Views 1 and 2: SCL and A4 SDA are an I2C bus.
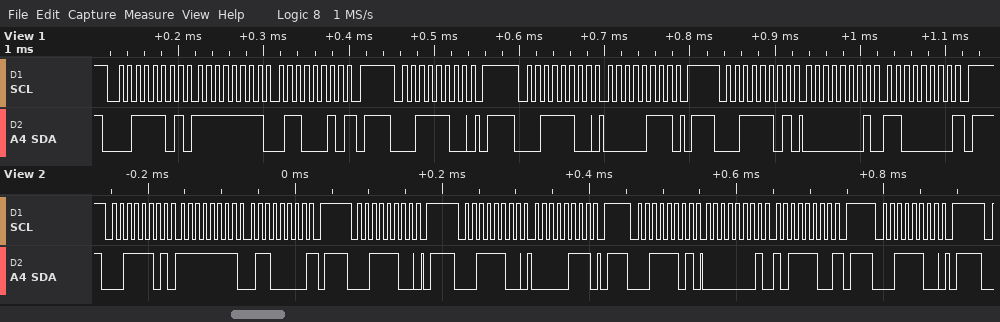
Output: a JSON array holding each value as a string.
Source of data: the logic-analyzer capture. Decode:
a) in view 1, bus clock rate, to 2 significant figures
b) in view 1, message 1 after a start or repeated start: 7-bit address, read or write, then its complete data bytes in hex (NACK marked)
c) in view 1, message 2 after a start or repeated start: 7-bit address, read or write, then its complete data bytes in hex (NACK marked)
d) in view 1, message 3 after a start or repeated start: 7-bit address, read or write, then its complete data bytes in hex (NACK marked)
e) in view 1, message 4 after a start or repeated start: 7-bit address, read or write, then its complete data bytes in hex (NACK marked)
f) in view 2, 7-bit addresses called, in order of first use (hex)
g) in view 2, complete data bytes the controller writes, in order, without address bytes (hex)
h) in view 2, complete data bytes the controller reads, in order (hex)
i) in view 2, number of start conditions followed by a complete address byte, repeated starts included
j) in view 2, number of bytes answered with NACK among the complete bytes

["100 kHz", "0x1E read: FF 62 NACK", "0x1E write", "0x1E write: 07", "0x1E read: 01 C0 NACK", "0x1E", "07", "FF 60 01 BC", "5", "2"]
